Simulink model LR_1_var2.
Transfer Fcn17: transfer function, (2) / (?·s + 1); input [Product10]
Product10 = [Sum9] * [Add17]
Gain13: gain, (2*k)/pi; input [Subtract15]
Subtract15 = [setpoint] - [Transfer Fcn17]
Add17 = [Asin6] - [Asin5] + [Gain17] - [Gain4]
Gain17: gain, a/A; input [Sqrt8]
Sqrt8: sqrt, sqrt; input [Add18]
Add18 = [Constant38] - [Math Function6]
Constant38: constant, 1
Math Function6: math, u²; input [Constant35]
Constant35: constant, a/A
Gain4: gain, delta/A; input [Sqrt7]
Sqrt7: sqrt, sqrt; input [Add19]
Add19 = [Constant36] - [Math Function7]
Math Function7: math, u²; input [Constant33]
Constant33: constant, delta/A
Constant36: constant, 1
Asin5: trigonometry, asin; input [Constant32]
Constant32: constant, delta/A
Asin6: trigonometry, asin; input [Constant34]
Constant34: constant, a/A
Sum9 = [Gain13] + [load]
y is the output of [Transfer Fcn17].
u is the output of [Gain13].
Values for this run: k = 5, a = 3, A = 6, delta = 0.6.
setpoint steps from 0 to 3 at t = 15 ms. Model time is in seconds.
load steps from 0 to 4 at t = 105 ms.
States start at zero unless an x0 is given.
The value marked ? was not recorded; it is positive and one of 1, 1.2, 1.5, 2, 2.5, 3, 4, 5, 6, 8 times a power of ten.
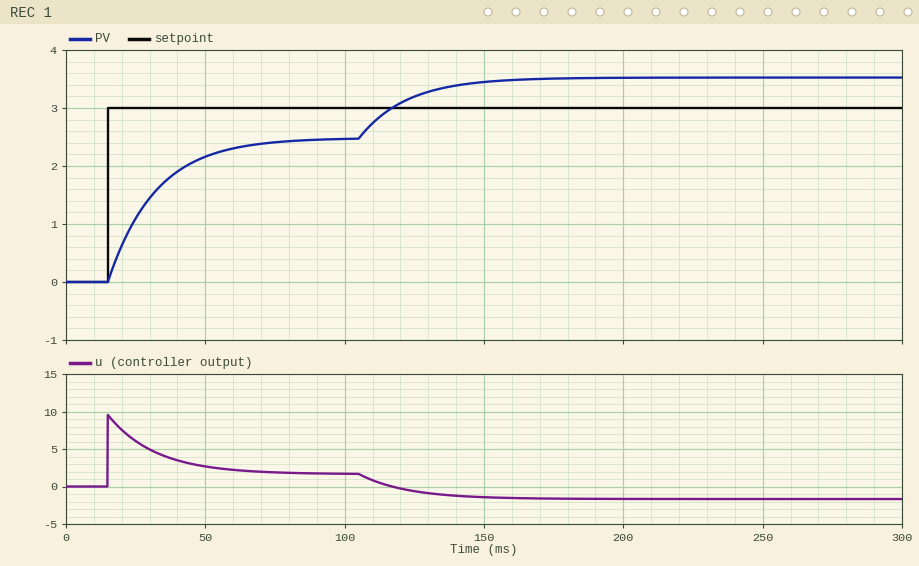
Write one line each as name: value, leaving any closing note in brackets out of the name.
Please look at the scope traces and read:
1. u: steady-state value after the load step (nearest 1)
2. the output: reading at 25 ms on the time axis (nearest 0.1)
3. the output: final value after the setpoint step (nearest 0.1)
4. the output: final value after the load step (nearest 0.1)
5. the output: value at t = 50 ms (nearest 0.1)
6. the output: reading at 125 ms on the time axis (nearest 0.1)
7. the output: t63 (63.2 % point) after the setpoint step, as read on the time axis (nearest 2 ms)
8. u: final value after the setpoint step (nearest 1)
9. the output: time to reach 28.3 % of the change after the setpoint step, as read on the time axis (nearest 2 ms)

u: steady-state value after the load step: -2
the output: reading at 25 ms on the time axis: 1.1
the output: final value after the setpoint step: 2.5
the output: final value after the load step: 3.5
the output: value at t = 50 ms: 2.2
the output: reading at 125 ms on the time axis: 3.2
the output: t63 (63.2 % point) after the setpoint step, as read on the time axis: 32 ms
u: final value after the setpoint step: 2
the output: time to reach 28.3 % of the change after the setpoint step, as read on the time axis: 20 ms
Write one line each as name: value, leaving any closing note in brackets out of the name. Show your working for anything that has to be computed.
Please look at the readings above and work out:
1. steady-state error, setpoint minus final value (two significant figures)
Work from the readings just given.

steady-state error, setpoint minus final value: 3 - 2.5 = 0.50
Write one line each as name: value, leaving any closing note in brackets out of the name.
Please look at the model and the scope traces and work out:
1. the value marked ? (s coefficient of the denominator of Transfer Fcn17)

the value marked ?: 0.1
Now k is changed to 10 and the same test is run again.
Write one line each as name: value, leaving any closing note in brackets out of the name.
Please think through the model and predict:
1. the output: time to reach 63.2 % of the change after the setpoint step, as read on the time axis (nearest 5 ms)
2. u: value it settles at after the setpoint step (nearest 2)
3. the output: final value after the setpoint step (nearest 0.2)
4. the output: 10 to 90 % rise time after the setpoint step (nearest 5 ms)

the output: time to reach 63.2 % of the change after the setpoint step, as read on the time axis: 25 ms
u: value it settles at after the setpoint step: 2
the output: final value after the setpoint step: 2.8
the output: 10 to 90 % rise time after the setpoint step: 20 ms
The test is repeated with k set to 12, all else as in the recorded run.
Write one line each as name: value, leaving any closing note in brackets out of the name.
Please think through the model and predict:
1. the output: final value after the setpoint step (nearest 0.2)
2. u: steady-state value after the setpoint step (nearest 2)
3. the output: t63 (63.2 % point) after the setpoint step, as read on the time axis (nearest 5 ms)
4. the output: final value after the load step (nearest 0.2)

the output: final value after the setpoint step: 2.8
u: steady-state value after the setpoint step: 2
the output: t63 (63.2 % point) after the setpoint step, as read on the time axis: 25 ms
the output: final value after the load step: 3.2
